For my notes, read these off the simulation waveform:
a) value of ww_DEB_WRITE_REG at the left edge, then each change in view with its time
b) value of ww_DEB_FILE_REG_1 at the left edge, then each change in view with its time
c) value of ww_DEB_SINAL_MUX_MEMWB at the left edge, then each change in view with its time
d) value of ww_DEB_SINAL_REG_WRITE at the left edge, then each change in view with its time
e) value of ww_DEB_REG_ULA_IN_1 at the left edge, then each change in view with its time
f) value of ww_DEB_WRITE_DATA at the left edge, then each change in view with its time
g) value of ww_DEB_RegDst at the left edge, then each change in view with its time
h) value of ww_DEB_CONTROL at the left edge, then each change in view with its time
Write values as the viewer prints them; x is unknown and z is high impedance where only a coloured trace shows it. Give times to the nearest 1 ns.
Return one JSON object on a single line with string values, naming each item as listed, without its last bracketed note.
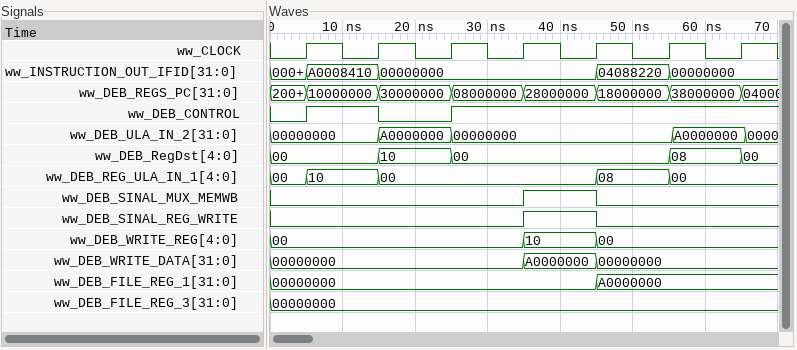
{"value of ww_DEB_WRITE_REG at the left edge, then each change in view with its time": "00, 10 at 35 ns, 00 at 45 ns", "value of ww_DEB_FILE_REG_1 at the left edge, then each change in view with its time": "00000000, A0000000 at 45 ns", "value of ww_DEB_SINAL_MUX_MEMWB at the left edge, then each change in view with its time": "0, 1 at 35 ns, 0 at 45 ns", "value of ww_DEB_SINAL_REG_WRITE at the left edge, then each change in view with its time": "0, 1 at 35 ns, 0 at 45 ns", "value of ww_DEB_REG_ULA_IN_1 at the left edge, then each change in view with its time": "00, 10 at 5 ns, 00 at 15 ns, 08 at 45 ns, 00 at 55 ns", "value of ww_DEB_WRITE_DATA at the left edge, then each change in view with its time": "00000000, A0000000 at 35 ns, 00000000 at 45 ns", "value of ww_DEB_RegDst at the left edge, then each change in view with its time": "00, 10 at 15 ns, 00 at 25 ns, 08 at 55 ns, 00 at 65 ns", "value of ww_DEB_CONTROL at the left edge, then each change in view with its time": "0, 1 at 5 ns, 0 at 15 ns, 1 at 25 ns"}
